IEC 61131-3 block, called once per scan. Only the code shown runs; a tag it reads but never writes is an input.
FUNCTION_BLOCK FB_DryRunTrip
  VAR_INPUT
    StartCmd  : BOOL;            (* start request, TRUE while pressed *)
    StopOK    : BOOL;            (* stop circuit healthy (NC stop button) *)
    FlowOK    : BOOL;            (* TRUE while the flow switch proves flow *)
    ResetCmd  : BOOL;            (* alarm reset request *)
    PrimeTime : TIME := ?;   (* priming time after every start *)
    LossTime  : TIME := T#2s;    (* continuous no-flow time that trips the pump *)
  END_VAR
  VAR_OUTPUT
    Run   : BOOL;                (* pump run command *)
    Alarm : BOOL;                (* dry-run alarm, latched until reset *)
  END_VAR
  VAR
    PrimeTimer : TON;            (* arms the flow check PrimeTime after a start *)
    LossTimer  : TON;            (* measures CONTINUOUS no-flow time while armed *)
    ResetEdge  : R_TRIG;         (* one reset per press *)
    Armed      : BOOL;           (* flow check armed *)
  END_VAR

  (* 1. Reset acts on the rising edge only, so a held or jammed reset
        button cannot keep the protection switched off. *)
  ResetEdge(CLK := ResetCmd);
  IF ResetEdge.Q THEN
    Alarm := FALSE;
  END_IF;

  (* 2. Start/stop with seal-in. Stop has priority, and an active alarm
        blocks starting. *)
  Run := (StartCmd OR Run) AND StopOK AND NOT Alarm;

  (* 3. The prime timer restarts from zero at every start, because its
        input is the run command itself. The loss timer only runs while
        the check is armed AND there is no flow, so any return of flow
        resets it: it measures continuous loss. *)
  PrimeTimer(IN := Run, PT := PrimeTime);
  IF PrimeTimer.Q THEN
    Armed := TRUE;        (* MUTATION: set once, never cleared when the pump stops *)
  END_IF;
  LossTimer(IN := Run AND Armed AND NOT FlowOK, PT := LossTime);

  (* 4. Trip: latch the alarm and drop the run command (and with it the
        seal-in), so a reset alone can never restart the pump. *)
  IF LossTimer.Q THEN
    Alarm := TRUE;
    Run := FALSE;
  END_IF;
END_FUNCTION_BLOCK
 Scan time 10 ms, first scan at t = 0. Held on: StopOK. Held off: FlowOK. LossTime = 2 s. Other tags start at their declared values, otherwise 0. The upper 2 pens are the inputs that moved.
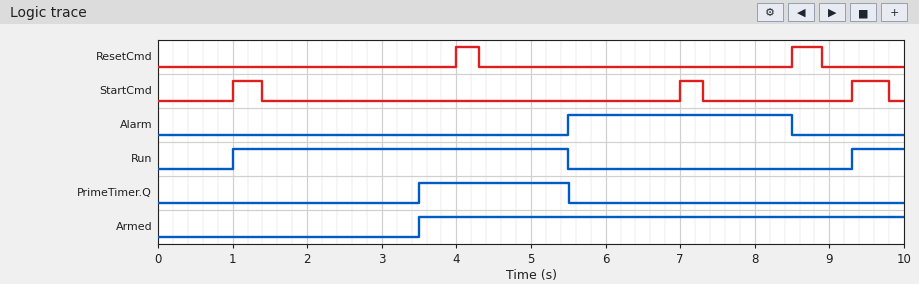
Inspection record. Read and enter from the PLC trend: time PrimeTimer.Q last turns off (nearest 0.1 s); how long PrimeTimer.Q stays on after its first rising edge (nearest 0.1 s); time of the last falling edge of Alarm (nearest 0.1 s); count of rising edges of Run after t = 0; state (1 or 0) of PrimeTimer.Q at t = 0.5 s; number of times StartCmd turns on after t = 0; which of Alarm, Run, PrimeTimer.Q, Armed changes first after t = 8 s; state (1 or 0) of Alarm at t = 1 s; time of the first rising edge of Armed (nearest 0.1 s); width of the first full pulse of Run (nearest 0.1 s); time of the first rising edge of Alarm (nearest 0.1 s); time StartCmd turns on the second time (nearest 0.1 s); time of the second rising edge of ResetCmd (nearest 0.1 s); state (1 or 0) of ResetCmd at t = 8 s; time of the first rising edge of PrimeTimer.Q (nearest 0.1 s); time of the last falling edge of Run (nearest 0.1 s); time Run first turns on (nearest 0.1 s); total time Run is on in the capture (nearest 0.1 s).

5.5 s
2.0 s
8.5 s
2
0
3
Alarm
0
3.5 s
4.5 s
5.5 s
7.0 s
8.5 s
0
3.5 s
5.5 s
1.0 s
5.2 s
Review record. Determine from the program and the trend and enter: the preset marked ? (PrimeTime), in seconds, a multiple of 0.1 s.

2.5 s
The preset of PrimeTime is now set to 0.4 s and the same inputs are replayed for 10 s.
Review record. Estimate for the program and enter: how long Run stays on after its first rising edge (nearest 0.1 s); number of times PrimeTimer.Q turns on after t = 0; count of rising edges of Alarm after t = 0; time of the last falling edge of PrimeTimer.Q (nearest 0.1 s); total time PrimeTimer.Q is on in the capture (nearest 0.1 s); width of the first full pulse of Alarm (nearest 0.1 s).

2.4 s
2
2
9.0 s
3.6 s
0.6 s
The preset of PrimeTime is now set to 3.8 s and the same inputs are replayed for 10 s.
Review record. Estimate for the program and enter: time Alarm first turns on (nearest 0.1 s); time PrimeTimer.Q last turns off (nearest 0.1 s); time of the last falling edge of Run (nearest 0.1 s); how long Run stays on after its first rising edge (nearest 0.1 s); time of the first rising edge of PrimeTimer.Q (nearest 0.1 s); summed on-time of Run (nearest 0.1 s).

6.8 s
6.8 s
6.8 s
5.8 s
4.8 s
6.5 s
